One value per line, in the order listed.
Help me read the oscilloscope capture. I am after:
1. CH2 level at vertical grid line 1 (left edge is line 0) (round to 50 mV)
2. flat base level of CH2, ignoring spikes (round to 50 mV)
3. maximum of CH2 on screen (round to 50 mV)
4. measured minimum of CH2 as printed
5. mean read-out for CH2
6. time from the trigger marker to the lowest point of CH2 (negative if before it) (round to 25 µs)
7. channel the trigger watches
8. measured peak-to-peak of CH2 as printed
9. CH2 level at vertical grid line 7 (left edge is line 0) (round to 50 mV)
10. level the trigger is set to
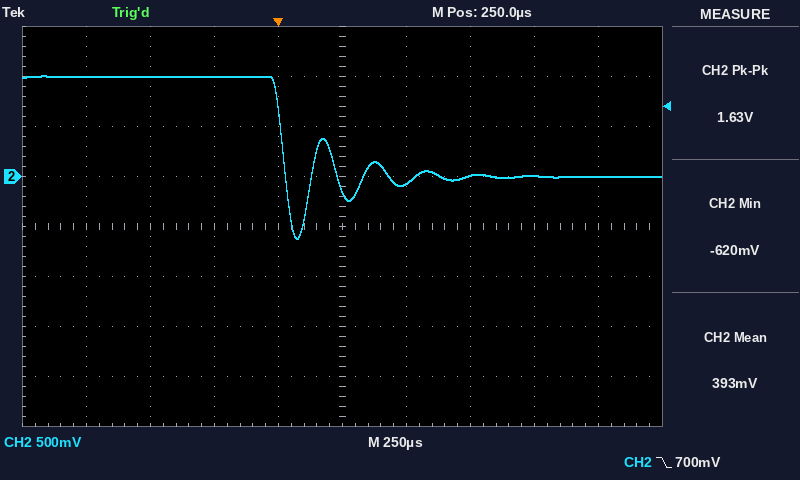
1.00 V
0 mV
1.00 V
-620 mV
393 mV
+75 µs
CH2
1.63 V
0 mV
700 mV
